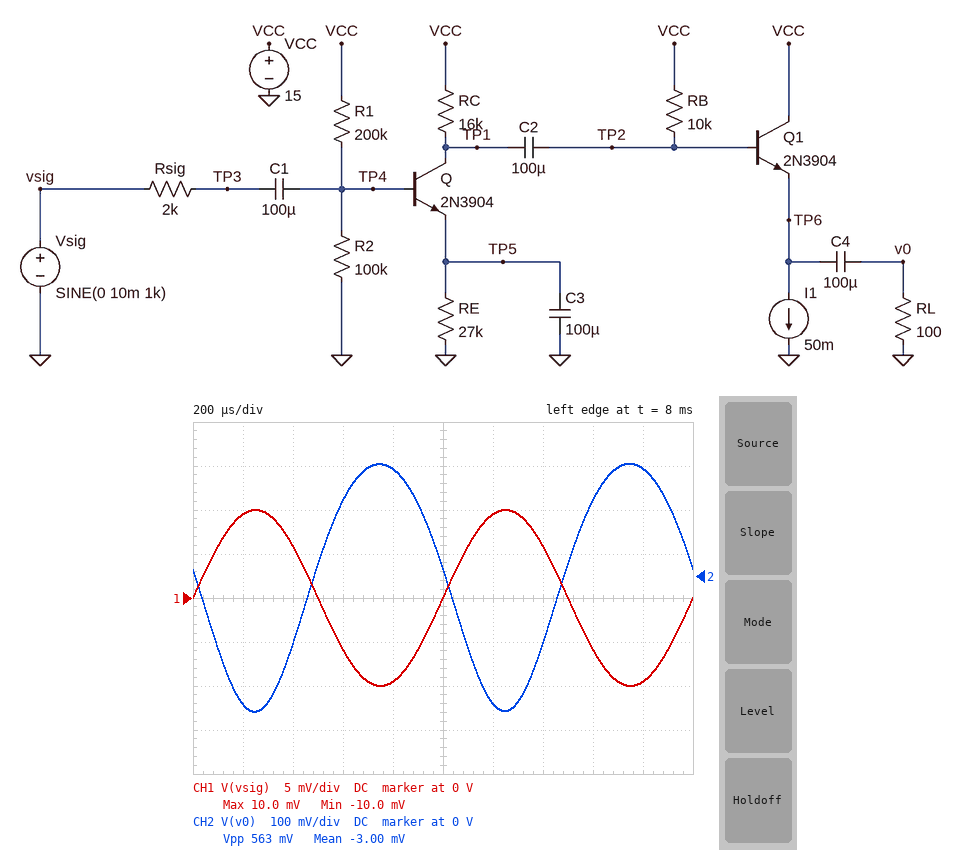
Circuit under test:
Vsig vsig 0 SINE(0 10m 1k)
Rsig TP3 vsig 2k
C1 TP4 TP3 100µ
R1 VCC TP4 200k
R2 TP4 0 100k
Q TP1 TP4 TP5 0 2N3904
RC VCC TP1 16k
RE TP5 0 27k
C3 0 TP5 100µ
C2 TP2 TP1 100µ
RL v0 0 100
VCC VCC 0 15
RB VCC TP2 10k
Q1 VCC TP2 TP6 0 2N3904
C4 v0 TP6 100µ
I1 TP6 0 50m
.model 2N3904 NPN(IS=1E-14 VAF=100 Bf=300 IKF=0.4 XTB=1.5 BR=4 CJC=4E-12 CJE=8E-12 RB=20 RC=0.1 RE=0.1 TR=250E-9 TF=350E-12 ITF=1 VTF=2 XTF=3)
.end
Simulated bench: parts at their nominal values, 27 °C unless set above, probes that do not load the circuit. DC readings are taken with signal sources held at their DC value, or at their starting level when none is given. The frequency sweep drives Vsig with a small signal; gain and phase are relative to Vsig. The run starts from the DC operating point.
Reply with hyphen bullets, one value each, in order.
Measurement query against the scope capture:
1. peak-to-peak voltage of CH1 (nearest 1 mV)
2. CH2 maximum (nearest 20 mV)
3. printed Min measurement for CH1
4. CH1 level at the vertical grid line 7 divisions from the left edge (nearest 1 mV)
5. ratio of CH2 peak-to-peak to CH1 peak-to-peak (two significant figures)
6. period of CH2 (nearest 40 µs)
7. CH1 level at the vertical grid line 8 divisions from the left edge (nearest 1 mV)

- 20 mV
- 260 mV
- -10.0 mV
- 6 mV
- 28
- 1.00 ms
- -6 mV
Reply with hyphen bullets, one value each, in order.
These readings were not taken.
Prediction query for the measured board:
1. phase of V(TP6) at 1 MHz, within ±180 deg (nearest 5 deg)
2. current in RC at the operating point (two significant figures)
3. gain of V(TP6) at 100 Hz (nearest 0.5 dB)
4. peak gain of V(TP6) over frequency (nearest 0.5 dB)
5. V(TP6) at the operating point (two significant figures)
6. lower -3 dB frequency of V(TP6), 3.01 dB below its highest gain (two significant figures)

- 130 deg
- 160 µA
- 29.0 dB
- 29.0 dB
- 12 V
- 7.0 Hz
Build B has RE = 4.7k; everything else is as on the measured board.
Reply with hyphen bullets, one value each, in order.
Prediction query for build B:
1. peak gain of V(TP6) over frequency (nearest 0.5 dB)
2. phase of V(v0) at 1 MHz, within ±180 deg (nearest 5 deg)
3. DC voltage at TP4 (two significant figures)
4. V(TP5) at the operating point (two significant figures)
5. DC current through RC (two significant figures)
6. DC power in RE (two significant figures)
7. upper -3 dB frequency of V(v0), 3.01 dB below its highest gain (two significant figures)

- -0.5 dB
- 95 deg
- 4.1 V
- 3.4 V
- 720 µA
- 2.5 mW
- 170 kHz
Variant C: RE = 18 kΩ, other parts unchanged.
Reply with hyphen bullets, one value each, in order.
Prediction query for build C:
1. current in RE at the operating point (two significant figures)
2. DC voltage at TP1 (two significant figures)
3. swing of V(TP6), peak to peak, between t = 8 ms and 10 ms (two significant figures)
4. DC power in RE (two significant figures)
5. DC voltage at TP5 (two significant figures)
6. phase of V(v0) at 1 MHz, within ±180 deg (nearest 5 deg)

- 240 µA
- 11 V
- 820 mV
- 1.0 mW
- 4.3 V
- 125 deg
